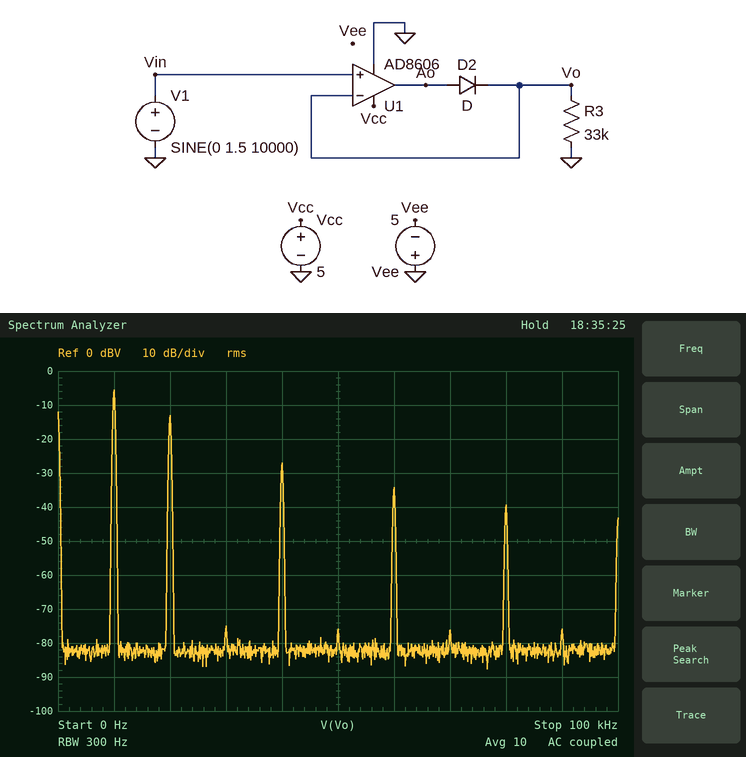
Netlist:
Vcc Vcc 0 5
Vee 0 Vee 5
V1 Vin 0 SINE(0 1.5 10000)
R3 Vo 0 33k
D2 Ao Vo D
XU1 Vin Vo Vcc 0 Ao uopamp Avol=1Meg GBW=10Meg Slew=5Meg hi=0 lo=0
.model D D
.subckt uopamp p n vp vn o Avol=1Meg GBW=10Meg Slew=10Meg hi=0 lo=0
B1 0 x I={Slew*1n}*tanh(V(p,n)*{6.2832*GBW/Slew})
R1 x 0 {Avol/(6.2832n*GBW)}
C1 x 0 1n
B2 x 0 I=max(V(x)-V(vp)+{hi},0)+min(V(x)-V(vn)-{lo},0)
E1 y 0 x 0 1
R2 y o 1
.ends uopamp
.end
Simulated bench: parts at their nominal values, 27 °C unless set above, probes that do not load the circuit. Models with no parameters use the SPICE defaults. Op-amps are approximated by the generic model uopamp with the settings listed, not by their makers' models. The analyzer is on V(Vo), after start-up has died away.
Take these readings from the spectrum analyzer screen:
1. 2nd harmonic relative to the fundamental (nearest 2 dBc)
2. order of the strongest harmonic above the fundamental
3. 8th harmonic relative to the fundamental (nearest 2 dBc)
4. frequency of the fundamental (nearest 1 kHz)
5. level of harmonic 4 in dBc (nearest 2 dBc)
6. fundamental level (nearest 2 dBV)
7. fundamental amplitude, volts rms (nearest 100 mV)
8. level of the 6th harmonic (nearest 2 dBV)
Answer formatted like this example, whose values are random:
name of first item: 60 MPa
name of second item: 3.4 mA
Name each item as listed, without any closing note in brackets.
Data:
2nd harmonic relative to the fundamental: -8 dBc
order of the strongest harmonic above the fundamental: 2
8th harmonic relative to the fundamental: -34 dBc
frequency of the fundamental: 10 kHz
level of harmonic 4 in dBc: -22 dBc
fundamental level: -6 dBV
fundamental amplitude, volts rms: 500 mV
level of the 6th harmonic: -34 dBV
